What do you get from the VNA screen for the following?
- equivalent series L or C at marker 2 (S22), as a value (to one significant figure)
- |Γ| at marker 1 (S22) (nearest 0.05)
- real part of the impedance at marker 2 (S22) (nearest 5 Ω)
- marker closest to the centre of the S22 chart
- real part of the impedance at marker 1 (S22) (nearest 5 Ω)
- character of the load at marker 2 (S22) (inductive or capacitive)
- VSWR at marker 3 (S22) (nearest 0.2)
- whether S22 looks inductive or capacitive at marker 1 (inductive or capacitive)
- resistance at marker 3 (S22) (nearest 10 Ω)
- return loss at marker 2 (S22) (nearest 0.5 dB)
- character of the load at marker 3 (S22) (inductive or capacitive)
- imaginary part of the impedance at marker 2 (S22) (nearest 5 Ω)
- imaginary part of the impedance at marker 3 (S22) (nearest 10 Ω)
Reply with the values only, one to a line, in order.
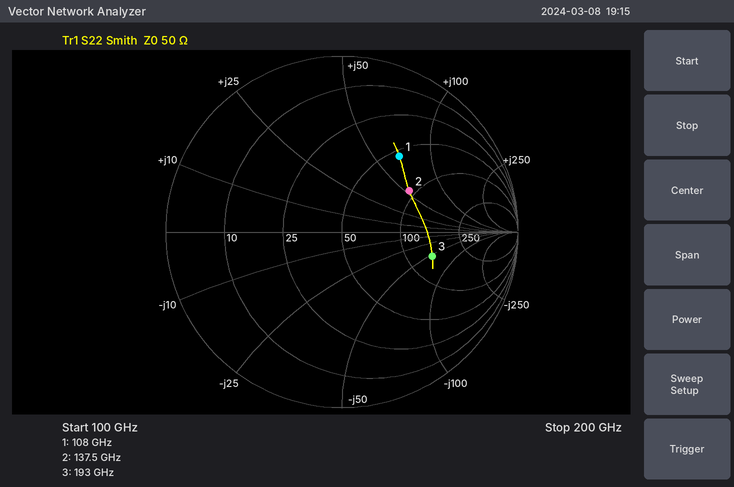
60 pH
0.55
90 Ω
marker 2
55 Ω
inductive
3.2
inductive
140 Ω
7.0 dB
capacitive
+55 Ω
-50 Ω
